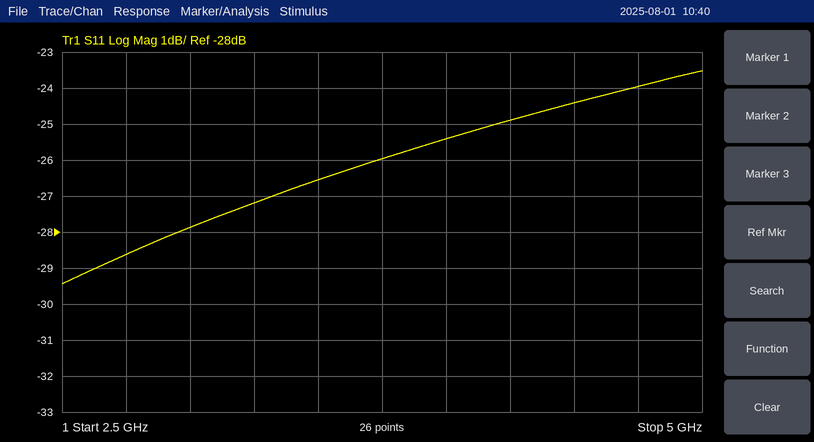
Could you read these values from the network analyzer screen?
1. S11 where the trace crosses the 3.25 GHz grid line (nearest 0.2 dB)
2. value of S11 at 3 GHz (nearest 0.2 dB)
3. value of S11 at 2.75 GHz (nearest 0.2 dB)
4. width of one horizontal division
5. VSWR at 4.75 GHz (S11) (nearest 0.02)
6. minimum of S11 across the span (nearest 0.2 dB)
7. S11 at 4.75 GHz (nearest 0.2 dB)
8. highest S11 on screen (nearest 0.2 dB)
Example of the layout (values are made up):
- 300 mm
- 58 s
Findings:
- -27.2 dB
- -27.8 dB
- -28.6 dB
- 250 MHz
- 1.14
- -29.4 dB
- -24.0 dB
- -23.6 dB
